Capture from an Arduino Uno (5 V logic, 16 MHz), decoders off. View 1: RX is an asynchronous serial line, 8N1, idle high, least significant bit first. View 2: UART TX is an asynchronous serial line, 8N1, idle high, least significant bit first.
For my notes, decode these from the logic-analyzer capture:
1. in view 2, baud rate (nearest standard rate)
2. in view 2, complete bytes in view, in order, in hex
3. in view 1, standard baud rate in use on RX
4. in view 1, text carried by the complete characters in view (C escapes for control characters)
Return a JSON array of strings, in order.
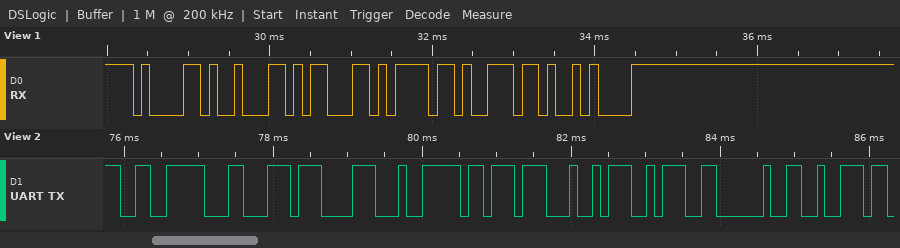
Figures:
["9600 baud", "0xE6 0x8C 0x87 0xE4 0xBB 0xA4 0x3A 0x20 0x72", "9600 baud", "\"abcon\\n\""]
